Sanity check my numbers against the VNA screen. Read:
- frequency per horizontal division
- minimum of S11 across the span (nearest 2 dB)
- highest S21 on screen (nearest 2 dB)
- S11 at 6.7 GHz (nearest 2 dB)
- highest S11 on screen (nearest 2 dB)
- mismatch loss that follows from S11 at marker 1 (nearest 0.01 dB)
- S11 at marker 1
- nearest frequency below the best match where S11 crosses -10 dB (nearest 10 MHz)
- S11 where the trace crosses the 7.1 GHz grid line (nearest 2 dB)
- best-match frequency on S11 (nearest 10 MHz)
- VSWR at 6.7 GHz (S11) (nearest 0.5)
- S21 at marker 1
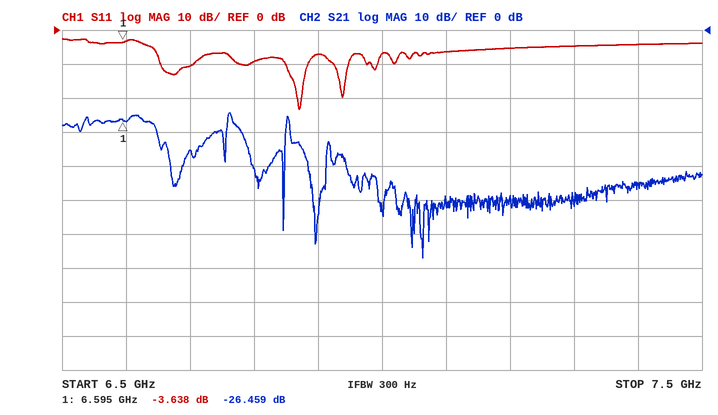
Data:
100 MHz
-24 dB
-24 dB
-10 dB
-2 dB
2.46 dB
-3.638 dB
6.85 GHz
-6 dB
6.87 GHz
2.0
-26.459 dB
